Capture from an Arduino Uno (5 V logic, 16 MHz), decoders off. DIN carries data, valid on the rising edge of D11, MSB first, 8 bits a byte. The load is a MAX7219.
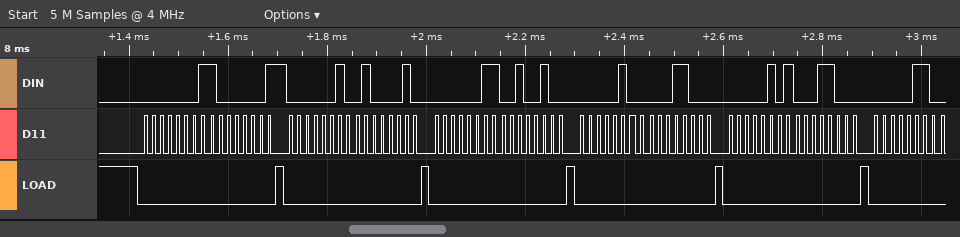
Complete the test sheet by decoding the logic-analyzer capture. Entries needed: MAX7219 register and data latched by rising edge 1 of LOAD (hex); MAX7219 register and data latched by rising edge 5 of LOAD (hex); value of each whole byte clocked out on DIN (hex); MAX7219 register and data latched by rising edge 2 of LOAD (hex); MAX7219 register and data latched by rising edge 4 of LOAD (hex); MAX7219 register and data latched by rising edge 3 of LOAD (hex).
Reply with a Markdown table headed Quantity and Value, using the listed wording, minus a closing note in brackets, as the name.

| Quantity | Value |
|---|---|
| MAX7219 register and data latched by rising edge 1 of LOAD | register 0x1, data 0x81 |
| MAX7219 register and data latched by rising edge 5 of LOAD | register 0x5, data 0x18 |
| value of each whole byte clocked out on DIN | 01 81 02 42 03 24 04 18 05 18 06 |
| MAX7219 register and data latched by rising edge 2 of LOAD | register 0x2, data 0x42 |
| MAX7219 register and data latched by rising edge 4 of LOAD | register 0x4, data 0x18 |
| MAX7219 register and data latched by rising edge 3 of LOAD | register 0x3, data 0x24 |
